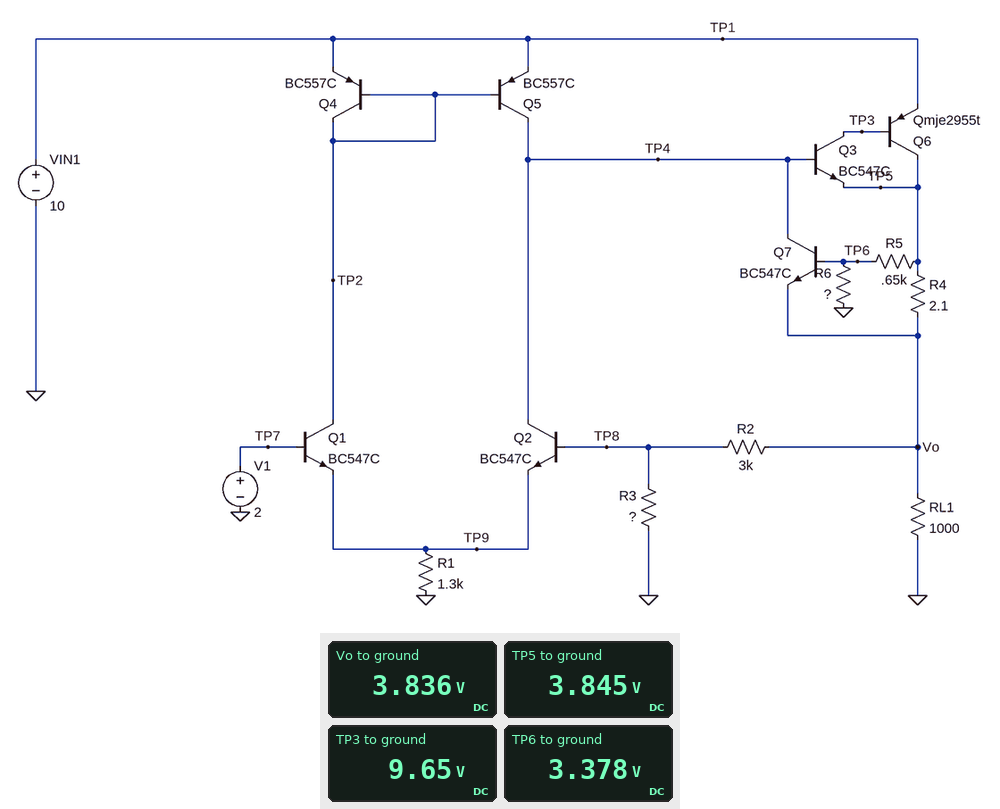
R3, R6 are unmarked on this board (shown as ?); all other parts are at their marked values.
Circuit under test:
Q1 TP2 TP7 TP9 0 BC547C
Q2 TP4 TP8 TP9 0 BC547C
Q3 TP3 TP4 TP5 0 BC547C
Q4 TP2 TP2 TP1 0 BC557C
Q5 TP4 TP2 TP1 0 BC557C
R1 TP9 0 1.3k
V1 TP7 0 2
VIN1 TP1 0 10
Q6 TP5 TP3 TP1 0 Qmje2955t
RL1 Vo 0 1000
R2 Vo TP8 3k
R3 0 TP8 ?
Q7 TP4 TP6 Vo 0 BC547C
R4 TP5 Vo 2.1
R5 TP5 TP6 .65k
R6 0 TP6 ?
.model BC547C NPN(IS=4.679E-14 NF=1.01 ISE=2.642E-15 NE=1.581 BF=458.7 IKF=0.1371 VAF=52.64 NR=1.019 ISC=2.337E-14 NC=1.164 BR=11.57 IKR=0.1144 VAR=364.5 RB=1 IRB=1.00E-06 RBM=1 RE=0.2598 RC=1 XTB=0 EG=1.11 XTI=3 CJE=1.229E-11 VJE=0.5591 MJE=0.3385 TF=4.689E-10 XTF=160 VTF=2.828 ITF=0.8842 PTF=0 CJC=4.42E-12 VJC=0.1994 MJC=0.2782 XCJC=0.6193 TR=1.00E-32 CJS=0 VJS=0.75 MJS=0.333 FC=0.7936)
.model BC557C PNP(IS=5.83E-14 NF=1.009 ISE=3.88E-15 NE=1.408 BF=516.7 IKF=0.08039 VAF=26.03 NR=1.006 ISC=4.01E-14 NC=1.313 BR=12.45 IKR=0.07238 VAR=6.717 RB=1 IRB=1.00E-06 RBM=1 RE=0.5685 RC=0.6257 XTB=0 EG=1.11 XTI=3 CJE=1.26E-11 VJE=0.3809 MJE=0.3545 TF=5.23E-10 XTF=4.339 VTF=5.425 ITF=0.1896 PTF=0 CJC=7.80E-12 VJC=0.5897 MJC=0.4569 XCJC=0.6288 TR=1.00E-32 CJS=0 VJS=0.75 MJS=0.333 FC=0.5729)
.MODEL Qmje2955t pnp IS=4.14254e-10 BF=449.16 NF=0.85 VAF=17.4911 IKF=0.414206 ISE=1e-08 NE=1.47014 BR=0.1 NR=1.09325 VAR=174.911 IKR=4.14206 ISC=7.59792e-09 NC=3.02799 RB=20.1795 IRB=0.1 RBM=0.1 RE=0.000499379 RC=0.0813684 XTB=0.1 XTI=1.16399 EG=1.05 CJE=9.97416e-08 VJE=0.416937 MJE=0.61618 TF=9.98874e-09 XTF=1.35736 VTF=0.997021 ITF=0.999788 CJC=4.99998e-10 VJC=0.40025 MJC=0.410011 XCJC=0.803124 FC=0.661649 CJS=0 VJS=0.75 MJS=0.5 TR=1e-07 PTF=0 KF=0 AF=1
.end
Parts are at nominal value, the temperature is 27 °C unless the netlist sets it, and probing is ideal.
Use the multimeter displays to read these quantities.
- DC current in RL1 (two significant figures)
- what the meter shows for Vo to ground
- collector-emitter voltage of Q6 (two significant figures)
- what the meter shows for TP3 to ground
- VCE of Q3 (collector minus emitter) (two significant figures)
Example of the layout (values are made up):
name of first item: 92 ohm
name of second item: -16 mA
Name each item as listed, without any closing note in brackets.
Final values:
DC current in RL1: 3.8 mA
what the meter shows for Vo to ground: 3.836 V
collector-emitter voltage of Q6: -6.2 V
what the meter shows for TP3 to ground: 9.65 V
VCE of Q3 (collector minus emitter): 5.8 V
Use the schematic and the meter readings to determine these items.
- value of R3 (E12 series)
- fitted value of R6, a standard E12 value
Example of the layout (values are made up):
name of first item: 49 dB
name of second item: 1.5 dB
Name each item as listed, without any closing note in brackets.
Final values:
value of R3: 3.3 kΩ
fitted value of R6, a standard E12 value: 4.7 kΩ
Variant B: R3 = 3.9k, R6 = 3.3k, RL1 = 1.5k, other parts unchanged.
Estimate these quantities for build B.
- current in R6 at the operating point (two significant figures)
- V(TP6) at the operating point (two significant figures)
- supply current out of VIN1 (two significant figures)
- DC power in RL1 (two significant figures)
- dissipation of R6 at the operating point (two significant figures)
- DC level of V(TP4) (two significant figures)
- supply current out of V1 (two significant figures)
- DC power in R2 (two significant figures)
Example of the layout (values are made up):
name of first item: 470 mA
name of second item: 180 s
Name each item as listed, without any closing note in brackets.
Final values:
current in R6 at the operating point: 900 µA
V(TP6) at the operating point: 3.0 V
supply current out of VIN1: 4.9 mA
DC power in RL1: 8.4 mW
dissipation of R6 at the operating point: 2.7 mW
DC level of V(TP4): 4.1 V
supply current out of V1: 940 nA
DC power in R2: 800 µW
